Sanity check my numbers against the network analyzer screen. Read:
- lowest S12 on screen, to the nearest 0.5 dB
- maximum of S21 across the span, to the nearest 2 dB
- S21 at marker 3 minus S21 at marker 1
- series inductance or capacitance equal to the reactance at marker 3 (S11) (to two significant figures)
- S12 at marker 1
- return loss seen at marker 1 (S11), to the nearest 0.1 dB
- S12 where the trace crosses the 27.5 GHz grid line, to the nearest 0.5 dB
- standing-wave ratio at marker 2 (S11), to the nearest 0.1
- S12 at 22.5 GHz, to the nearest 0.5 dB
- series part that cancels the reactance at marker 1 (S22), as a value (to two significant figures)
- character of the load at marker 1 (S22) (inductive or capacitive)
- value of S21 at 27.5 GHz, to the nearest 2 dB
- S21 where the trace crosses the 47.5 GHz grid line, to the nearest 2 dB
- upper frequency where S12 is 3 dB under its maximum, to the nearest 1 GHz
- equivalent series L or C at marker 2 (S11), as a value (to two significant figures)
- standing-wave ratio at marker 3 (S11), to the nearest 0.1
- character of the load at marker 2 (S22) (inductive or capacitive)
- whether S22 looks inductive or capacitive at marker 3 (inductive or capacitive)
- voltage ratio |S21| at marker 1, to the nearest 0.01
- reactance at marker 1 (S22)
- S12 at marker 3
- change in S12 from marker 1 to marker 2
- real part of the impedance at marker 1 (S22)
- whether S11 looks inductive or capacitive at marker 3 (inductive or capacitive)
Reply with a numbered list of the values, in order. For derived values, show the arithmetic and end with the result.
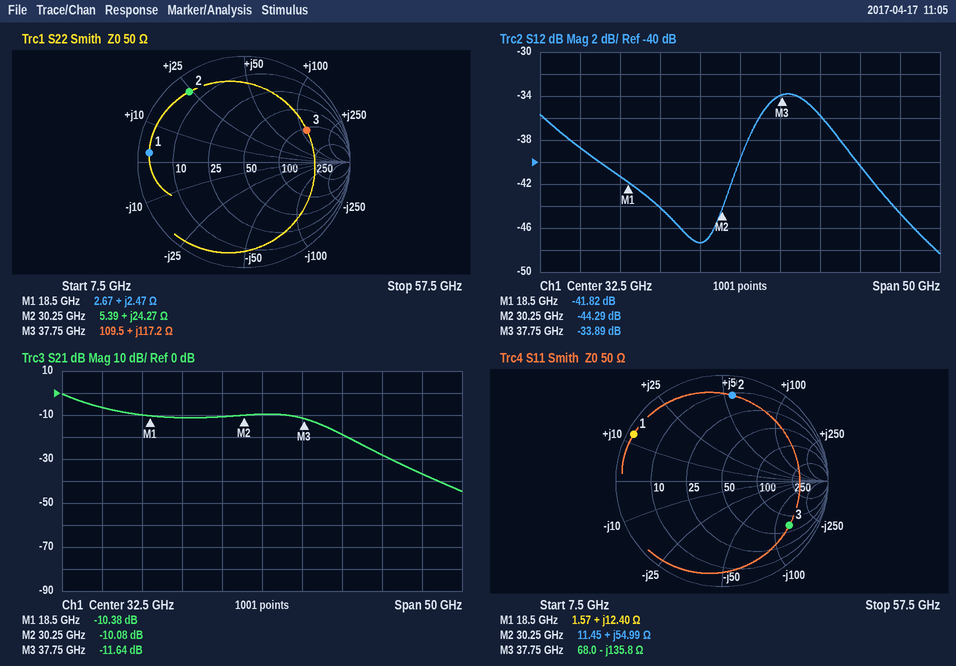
1. -48.5 dB
2. 0 dB
3. -11.64 − (-10.38) = -1.26 dB
4. C = 1/(2π × 37.75 GHz × 135.8 Ω) ≈ 31 fF
5. -41.82 dB
6. 0.5 dB
7. -47.5 dB
8. 9.8
9. -44.0 dB
10. C = 1/(2π × 18.5 GHz × 2.47 Ω) ≈ 3.5 pF
11. inductive
12. -10 dB
13. -28 dB
14. 44 GHz
15. L = 54.99 Ω/(2π × 30.25 GHz) ≈ 289 pH, so 290 pH to two significant figures
16. 7.4
17. inductive
18. inductive
19. 10^(-10.38/20) ≈ 0.30
20. +2.47 Ω
21. -33.89 dB
22. -44.29 − (-41.82) = -2.47 dB
23. 2.67 Ω
24. capacitive
